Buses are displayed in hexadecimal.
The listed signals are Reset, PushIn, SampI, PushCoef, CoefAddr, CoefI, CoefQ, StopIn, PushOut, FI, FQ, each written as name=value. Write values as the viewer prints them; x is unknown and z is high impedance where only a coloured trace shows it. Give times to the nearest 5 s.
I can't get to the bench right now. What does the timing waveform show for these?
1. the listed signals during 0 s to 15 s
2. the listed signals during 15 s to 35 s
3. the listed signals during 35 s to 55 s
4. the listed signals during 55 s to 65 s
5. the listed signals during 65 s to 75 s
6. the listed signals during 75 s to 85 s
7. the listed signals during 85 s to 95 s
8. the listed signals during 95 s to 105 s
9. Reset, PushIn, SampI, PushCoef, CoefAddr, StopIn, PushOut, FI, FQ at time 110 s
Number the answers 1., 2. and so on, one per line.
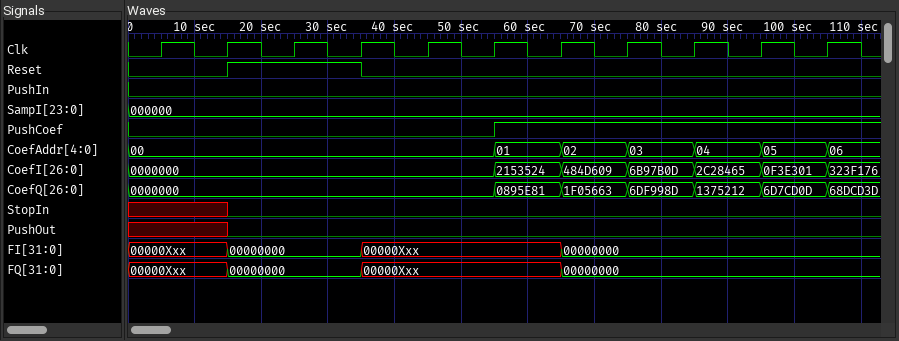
1. Reset=0, PushIn=0, SampI=000000, PushCoef=0, CoefAddr=00, CoefI=0000000, CoefQ=0000000, StopIn=x, PushOut=x, FI=00000Xxx, FQ=00000Xxx
2. Reset=1, PushIn=0, SampI=000000, PushCoef=0, CoefAddr=00, CoefI=0000000, CoefQ=0000000, StopIn=0, PushOut=0, FI=00000000, FQ=00000000
3. Reset=0, PushIn=0, SampI=000000, PushCoef=0, CoefAddr=00, CoefI=0000000, CoefQ=0000000, StopIn=0, PushOut=0, FI=00000Xxx, FQ=00000Xxx
4. Reset=0, PushIn=0, SampI=000000, PushCoef=1, CoefAddr=01, CoefI=2153524, CoefQ=0895E81, StopIn=0, PushOut=0, FI=00000Xxx, FQ=00000Xxx
5. Reset=0, PushIn=0, SampI=000000, PushCoef=1, CoefAddr=02, CoefI=484D609, CoefQ=1F05663, StopIn=0, PushOut=0, FI=00000000, FQ=00000000
6. Reset=0, PushIn=0, SampI=000000, PushCoef=1, CoefAddr=03, CoefI=6B97B0D, CoefQ=6DF998D, StopIn=0, PushOut=0, FI=00000000, FQ=00000000
7. Reset=0, PushIn=0, SampI=000000, PushCoef=1, CoefAddr=04, CoefI=2C28465, CoefQ=1375212, StopIn=0, PushOut=0, FI=00000000, FQ=00000000
8. Reset=0, PushIn=0, SampI=000000, PushCoef=1, CoefAddr=05, CoefI=0F3E301, CoefQ=6D7CD0D, StopIn=0, PushOut=0, FI=00000000, FQ=00000000
9. Reset=0, PushIn=0, SampI=000000, PushCoef=1, CoefAddr=06, StopIn=0, PushOut=0, FI=00000000, FQ=00000000
